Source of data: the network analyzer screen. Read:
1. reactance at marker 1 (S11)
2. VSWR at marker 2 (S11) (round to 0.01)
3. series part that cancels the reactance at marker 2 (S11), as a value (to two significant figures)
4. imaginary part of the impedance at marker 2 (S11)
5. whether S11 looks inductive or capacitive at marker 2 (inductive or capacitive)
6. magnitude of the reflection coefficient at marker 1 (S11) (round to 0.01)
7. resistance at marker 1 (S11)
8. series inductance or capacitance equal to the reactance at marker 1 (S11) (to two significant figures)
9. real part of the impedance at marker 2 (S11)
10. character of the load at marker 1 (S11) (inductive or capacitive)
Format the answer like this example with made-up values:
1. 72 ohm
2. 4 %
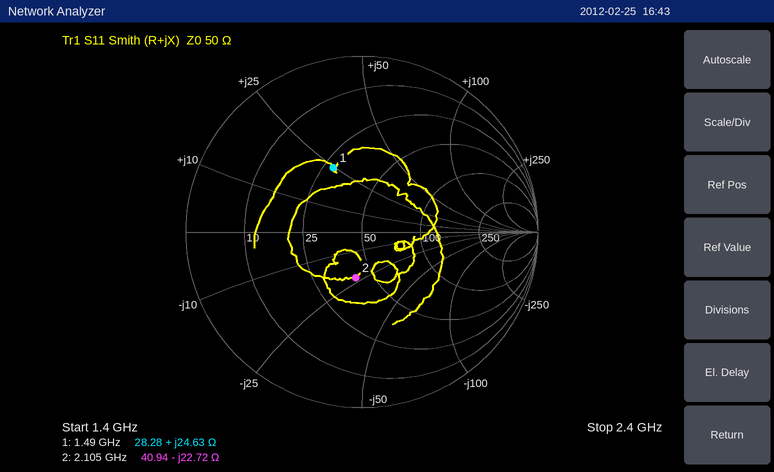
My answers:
1. +24.63 Ω
2. 1.71
3. 1.7 nH
4. -22.72 Ω
5. capacitive
6. 0.40
7. 28.28 Ω
8. 2.6 nH
9. 40.94 Ω
10. inductive
